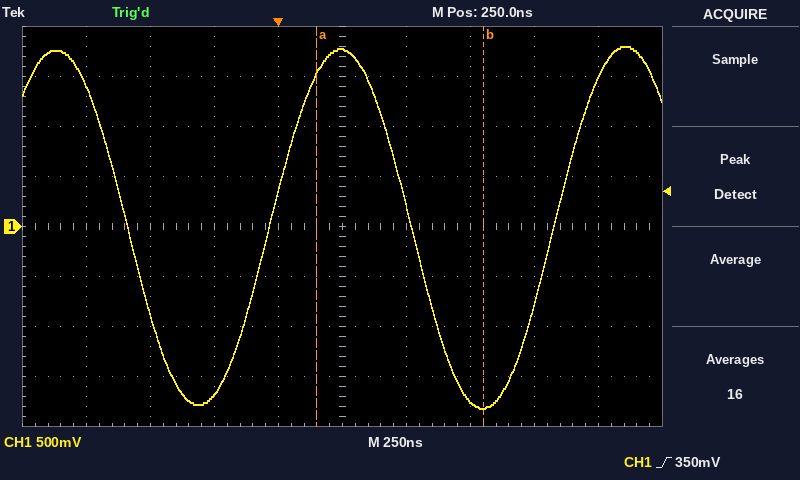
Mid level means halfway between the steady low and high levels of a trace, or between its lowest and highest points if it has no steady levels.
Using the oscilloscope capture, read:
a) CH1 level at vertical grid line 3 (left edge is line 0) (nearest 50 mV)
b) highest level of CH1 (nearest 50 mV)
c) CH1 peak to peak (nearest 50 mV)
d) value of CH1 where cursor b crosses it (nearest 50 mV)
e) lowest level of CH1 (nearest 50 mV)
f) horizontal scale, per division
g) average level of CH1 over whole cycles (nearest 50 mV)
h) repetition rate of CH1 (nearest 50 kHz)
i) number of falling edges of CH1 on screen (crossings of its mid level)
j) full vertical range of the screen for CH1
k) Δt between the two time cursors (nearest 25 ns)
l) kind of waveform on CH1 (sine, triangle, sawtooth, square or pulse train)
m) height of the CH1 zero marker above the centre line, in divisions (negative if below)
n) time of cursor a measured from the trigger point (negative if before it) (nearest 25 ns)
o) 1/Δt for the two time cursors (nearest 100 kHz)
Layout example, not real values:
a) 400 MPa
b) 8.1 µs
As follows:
a) -1.70 V
b) 1.80 V
c) 3.60 V
d) -1.80 V
e) -1.80 V
f) 250 ns
g) 0 mV
h) 900 kHz
i) 2
j) 4 V
k) 650 ns
l) sine
m) 0.0 div
n) +150 ns
o) 1.5 MHz
